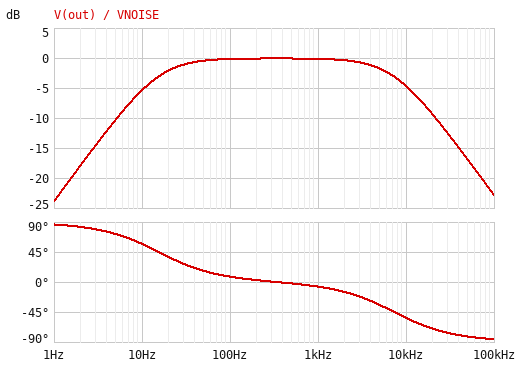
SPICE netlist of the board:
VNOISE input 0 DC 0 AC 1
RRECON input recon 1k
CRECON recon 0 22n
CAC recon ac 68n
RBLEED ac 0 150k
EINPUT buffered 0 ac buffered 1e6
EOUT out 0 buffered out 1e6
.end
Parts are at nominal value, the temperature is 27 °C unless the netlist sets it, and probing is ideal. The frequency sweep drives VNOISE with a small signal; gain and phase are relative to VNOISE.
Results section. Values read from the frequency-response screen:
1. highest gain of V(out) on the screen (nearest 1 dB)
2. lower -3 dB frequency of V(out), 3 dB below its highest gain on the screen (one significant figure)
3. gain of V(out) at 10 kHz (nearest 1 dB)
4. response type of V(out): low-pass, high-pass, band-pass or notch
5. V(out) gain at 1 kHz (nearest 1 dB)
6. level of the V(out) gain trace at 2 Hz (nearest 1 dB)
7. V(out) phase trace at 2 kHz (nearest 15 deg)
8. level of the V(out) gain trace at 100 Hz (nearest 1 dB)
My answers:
0 dB
20 Hz
-5 dB
band-pass
0 dB
-18 dB
-15 deg
0 dB
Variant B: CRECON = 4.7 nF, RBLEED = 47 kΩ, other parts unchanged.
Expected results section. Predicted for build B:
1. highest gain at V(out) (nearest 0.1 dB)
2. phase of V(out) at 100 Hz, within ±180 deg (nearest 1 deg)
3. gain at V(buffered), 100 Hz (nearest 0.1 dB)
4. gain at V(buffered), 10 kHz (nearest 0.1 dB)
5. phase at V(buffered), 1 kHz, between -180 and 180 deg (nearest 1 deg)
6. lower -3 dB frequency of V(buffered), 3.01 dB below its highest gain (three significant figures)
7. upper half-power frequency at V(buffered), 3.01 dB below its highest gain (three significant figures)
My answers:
-0.2 dB
26 deg
-1.1 dB
-0.5 dB
1 deg
48.6 Hz
34.7 kHz
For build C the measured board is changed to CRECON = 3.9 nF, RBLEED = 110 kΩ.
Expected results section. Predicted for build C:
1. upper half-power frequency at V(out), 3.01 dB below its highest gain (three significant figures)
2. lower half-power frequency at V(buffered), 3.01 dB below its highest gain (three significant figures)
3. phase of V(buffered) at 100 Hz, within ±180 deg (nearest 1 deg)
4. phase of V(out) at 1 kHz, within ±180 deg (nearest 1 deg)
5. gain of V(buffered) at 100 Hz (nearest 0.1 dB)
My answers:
41.2 kHz
21.1 Hz
12 deg
0 deg
-0.3 dB
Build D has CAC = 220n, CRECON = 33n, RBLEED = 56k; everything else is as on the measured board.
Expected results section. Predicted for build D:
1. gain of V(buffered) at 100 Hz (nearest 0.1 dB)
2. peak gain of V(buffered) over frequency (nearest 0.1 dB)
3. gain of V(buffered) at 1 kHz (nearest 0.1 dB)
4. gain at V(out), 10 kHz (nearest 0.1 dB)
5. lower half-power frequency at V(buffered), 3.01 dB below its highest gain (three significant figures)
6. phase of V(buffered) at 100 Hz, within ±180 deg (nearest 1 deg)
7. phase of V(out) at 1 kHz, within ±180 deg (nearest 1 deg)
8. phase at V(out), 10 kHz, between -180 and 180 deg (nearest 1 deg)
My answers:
-0.2 dB
-0.2 dB
-0.3 dB
-7.3 dB
12.6 Hz
6 deg
-11 deg
-64 deg
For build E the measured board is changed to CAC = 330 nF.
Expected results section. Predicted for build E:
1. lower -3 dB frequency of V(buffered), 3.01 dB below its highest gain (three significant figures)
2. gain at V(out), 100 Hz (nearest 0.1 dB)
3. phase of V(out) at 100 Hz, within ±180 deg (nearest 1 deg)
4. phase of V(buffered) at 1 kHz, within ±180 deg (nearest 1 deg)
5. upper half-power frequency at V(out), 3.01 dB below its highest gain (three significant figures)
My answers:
3.19 Hz
-0.1 dB
1 deg
-8 deg
7.29 kHz
